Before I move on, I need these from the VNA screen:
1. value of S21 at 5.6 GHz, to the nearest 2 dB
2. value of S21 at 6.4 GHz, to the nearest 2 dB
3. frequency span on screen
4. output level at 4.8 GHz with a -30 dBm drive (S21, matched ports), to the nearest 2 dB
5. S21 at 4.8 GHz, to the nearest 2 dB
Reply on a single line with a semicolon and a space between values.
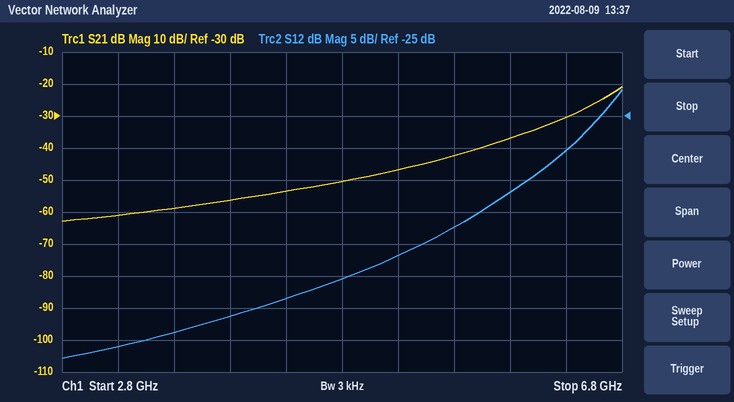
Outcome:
-42 dB; -30 dB; 4 GHz; -80 dBm; -50 dB
